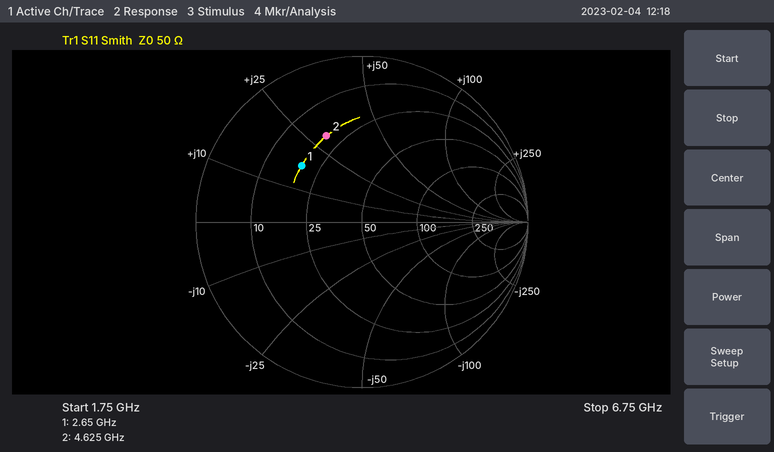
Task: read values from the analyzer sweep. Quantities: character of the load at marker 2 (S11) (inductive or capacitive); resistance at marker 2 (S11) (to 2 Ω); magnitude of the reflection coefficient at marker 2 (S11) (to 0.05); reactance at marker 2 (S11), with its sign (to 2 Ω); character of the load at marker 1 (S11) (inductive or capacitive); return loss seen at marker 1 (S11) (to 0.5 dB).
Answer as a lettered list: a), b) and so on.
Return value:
a) inductive
b) 20 Ω
c) 0.55
d) +30 Ω
e) inductive
f) 6.0 dB
